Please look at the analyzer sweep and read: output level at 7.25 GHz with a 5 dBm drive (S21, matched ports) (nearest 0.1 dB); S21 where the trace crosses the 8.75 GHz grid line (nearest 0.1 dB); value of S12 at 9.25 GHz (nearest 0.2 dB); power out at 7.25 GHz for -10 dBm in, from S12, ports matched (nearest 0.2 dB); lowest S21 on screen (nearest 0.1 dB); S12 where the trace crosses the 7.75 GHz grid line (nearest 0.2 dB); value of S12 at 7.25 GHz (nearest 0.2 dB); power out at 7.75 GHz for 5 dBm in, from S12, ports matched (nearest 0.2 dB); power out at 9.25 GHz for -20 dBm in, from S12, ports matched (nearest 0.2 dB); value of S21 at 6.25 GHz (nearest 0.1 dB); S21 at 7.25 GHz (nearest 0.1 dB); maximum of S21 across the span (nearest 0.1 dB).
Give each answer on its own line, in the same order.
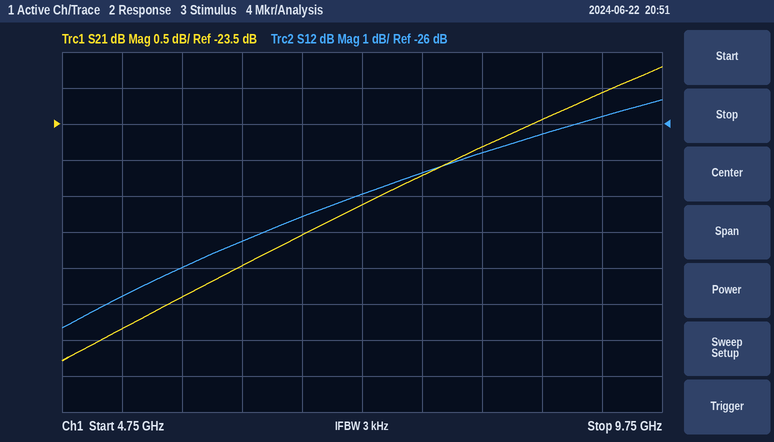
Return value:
-19.6 dBm
-23.4 dB
-25.8 dB
-38.0 dBm
-26.8 dB
-27.4 dB
-28.0 dB
-22.4 dBm
-45.8 dBm
-25.5 dB
-24.6 dB
-22.7 dB
